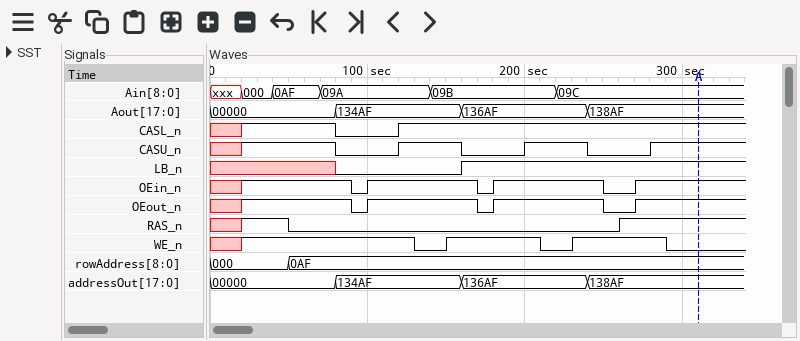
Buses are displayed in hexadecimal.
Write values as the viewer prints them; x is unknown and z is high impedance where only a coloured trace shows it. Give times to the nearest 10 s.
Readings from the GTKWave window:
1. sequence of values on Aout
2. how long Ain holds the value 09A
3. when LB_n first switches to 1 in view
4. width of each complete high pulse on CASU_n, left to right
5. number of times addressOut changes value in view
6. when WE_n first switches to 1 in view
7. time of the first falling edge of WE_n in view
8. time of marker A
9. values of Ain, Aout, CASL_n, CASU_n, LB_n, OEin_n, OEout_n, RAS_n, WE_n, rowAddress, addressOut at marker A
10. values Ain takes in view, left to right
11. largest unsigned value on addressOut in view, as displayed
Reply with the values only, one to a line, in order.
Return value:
00000, 134AF, 136AF, 138AF
70 s
160 s
40 s, 40 s
3
20 s
130 s
310 s
Ain=09C, Aout=138AF, CASL_n=1, CASU_n=1, LB_n=1, OEin_n=1, OEout_n=1, RAS_n=1, WE_n=0, rowAddress=0AF, addressOut=138AF
xxx, 000, 0AF, 09A, 09B, 09C
138AF
